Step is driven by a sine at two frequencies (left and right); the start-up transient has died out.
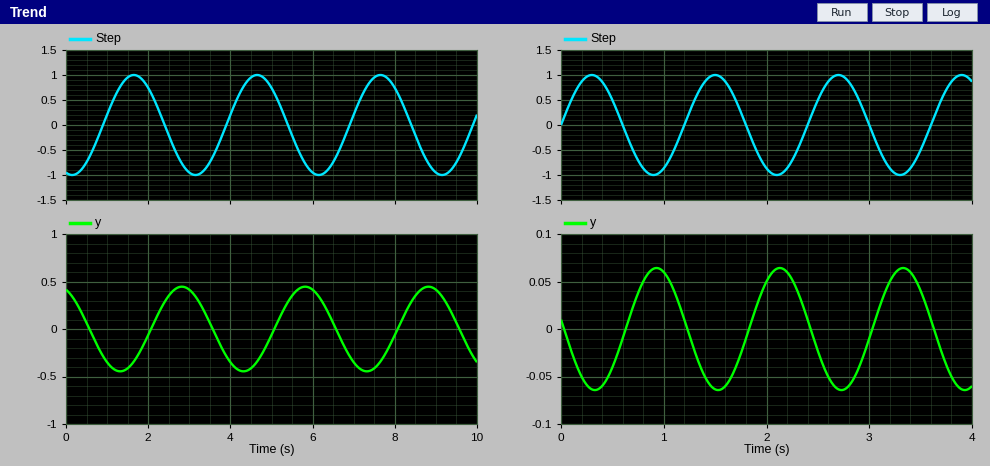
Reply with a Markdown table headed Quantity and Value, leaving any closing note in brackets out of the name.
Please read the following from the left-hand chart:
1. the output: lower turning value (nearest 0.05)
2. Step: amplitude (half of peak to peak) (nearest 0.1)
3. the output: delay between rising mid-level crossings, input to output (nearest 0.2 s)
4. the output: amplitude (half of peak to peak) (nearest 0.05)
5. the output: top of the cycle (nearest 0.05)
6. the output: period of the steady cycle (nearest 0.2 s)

| Quantity | Value |
|---|---|
| the output: lower turning value | -0.45 |
| Step: amplitude (half of peak to peak) | 1.0 |
| the output: delay between rising mid-level crossings, input to output | 1.2 s |
| the output: amplitude (half of peak to peak) | 0.45 |
| the output: top of the cycle | 0.45 |
| the output: period of the steady cycle | 3.0 s |
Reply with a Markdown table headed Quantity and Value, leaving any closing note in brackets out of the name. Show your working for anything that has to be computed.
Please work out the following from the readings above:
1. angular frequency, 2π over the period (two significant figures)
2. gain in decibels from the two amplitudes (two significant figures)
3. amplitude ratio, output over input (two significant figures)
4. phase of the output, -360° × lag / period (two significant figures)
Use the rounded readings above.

| Quantity | Value |
|---|---|
| angular frequency, 2π over the period | 2π / 3 = 2.1 rad/s |
| gain in decibels from the two amplitudes | 20 log10(0.45 / 1) = -6.9 dB |
| amplitude ratio, output over input | 0.45 / 1 = 0.45 |
| phase of the output, -360° × lag / period | -360 × 1.2 / 3 = -140° |
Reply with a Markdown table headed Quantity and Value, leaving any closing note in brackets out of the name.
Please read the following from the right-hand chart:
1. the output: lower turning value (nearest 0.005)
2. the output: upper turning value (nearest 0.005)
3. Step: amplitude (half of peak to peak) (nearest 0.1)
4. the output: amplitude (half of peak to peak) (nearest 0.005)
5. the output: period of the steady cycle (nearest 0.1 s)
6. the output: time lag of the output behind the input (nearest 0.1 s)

| Quantity | Value |
|---|---|
| the output: lower turning value | -0.065 |
| the output: upper turning value | 0.065 |
| Step: amplitude (half of peak to peak) | 1.0 |
| the output: amplitude (half of peak to peak) | 0.065 |
| the output: period of the steady cycle | 1.2 s |
| the output: time lag of the output behind the input | 0.6 s |
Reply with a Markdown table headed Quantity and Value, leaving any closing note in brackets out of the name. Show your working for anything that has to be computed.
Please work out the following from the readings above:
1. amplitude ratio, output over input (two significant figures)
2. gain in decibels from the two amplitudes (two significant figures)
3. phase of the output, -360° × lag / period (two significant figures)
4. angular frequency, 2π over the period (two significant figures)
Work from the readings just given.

| Quantity | Value |
|---|---|
| amplitude ratio, output over input | 0.065 / 1 = 0.065 |
| gain in decibels from the two amplitudes | 20 log10(0.065 / 1) = -24 dB |
| phase of the output, -360° × lag / period | -360 × 0.6 / 1.2 = -180° |
| angular frequency, 2π over the period | 2π / 1.2 = 5.2 rad/s |
